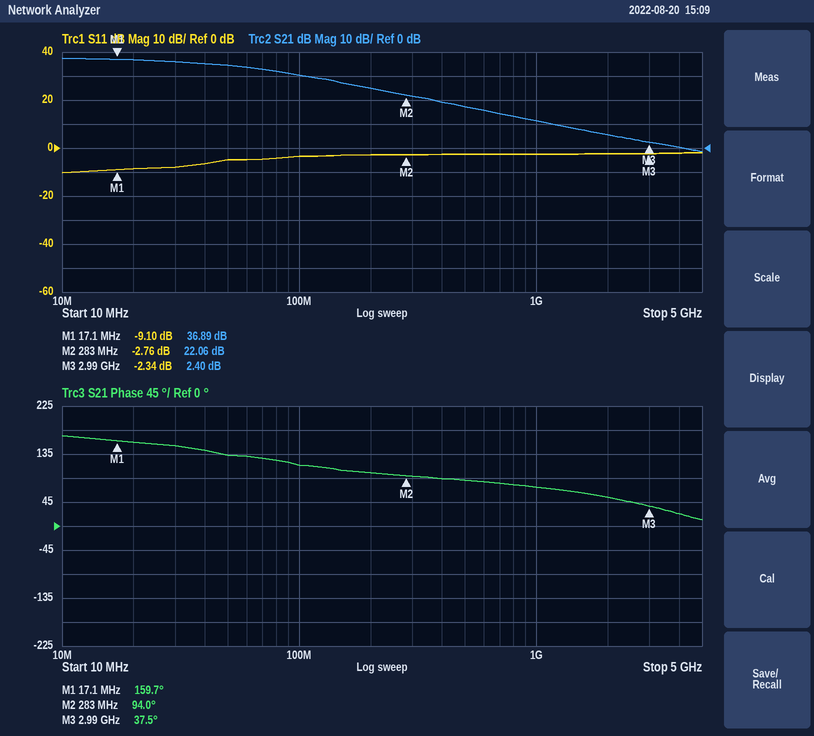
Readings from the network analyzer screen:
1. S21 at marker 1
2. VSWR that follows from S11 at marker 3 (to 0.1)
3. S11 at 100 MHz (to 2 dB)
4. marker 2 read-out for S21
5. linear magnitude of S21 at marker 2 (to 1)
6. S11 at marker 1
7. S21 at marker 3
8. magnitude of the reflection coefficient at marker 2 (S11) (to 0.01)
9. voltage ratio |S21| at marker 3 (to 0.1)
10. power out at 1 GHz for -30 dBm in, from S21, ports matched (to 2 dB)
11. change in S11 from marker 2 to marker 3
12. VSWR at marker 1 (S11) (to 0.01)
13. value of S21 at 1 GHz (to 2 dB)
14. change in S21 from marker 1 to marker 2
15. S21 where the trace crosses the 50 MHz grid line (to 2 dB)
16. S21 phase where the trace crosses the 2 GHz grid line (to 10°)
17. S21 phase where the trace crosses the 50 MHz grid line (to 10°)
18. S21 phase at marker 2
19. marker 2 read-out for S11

36.89 dB
7.5
-4 dB
22.06 dB
13
-9.10 dB
2.40 dB
0.73
1.3
-18 dBm
0.42 dB
2.08
12 dB
-14.83 dB
34 dB
50°
130°
94.0°
-2.76 dB
